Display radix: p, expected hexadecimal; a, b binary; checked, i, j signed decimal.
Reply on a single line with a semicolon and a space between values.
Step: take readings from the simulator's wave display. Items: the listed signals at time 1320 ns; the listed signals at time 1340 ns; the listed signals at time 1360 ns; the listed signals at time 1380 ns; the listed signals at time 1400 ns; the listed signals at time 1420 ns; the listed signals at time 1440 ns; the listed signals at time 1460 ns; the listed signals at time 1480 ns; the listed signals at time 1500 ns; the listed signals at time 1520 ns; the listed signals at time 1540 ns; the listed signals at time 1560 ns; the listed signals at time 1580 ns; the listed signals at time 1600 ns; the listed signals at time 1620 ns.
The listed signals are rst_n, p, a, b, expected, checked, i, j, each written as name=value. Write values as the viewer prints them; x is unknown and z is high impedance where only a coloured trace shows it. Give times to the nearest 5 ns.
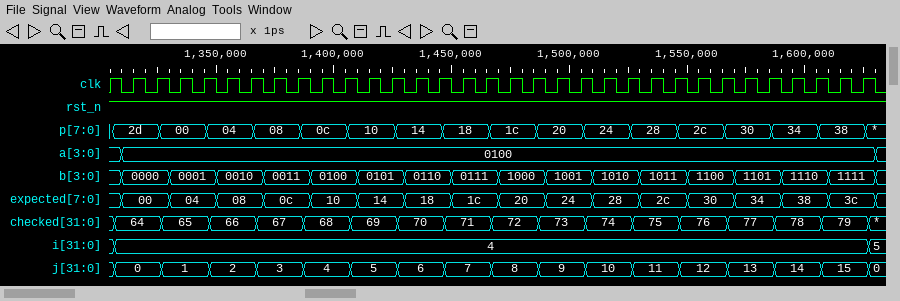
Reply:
rst_n=1, p=2d, a=0100, b=0000, expected=00, checked=64, i=4, j=0; rst_n=1, p=00, a=0100, b=0001, expected=04, checked=65, i=4, j=1; rst_n=1, p=04, a=0100, b=0010, expected=08, checked=66, i=4, j=2; rst_n=1, p=08, a=0100, b=0011, expected=0c, checked=67, i=4, j=3; rst_n=1, p=0c, a=0100, b=0100, expected=10, checked=68, i=4, j=4; rst_n=1, p=10, a=0100, b=0101, expected=14, checked=69, i=4, j=5; rst_n=1, p=14, a=0100, b=0110, expected=18, checked=70, i=4, j=6; rst_n=1, p=18, a=0100, b=0111, expected=1c, checked=71, i=4, j=7; rst_n=1, p=1c, a=0100, b=1000, expected=20, checked=72, i=4, j=8; rst_n=1, p=20, a=0100, b=1001, expected=24, checked=73, i=4, j=9; rst_n=1, p=24, a=0100, b=1010, expected=28, checked=74, i=4, j=10; rst_n=1, p=28, a=0100, b=1011, expected=2c, checked=75, i=4, j=11; rst_n=1, p=2c, a=0100, b=1100, expected=30, checked=76, i=4, j=12; rst_n=1, p=30, a=0100, b=1101, expected=34, checked=77, i=4, j=13; rst_n=1, p=34, a=0100, b=1110, expected=38, checked=78, i=4, j=14; rst_n=1, p=38, a=0100, b=1111, expected=3c, checked=79, i=4, j=15
